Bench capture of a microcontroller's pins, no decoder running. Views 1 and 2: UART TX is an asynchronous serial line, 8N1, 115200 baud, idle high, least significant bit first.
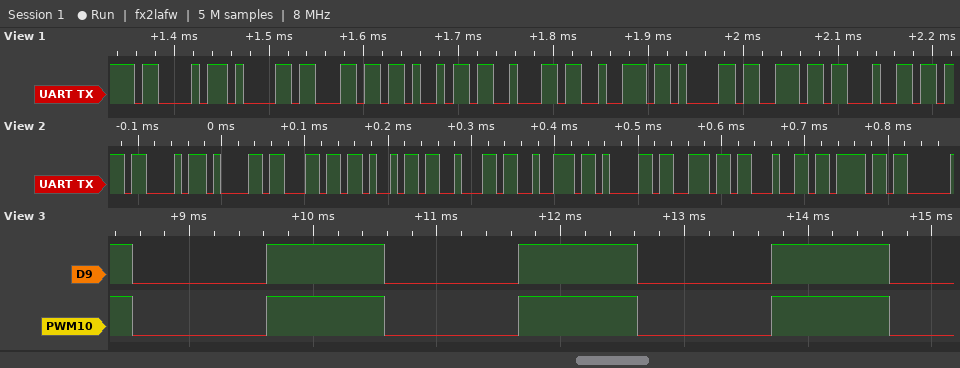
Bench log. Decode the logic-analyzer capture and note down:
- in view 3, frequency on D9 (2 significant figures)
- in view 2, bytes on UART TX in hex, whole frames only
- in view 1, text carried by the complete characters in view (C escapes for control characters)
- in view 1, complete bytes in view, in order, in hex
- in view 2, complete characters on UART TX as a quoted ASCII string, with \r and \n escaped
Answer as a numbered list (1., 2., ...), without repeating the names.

1. 490 Hz
2. 0x43 0x61 0x6C 0x69 0x62 0x72 0x61 0x6E 0x64 0x6F
3. "Calibrand"
4. 43 61 6C 69 62 72 61 6E 64
5. "Calibrando"
